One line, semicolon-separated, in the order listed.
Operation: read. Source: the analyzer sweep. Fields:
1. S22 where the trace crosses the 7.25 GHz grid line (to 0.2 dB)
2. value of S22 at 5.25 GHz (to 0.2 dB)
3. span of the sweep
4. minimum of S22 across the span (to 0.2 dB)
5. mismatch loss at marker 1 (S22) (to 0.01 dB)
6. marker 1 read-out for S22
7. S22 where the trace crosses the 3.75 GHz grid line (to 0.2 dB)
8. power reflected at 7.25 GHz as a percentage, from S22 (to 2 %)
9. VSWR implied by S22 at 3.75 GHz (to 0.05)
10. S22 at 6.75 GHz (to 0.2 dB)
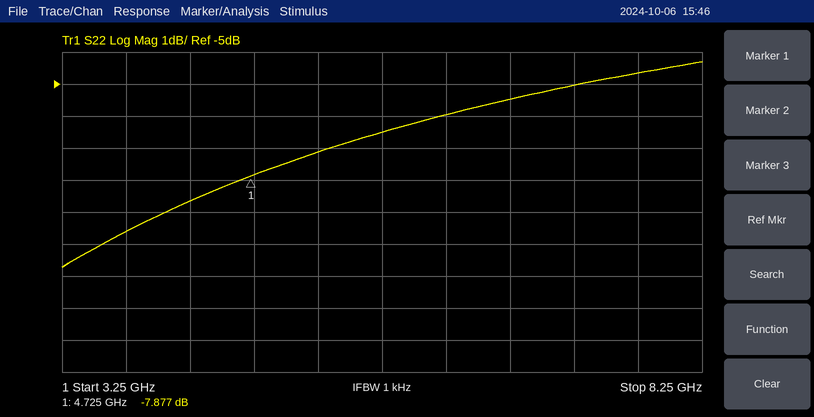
-5.0 dB; -7.2 dB; 5 GHz; -10.8 dB; 0.77 dB; -7.877 dB; -9.6 dB; 32 %; 2.00; -5.4 dB
